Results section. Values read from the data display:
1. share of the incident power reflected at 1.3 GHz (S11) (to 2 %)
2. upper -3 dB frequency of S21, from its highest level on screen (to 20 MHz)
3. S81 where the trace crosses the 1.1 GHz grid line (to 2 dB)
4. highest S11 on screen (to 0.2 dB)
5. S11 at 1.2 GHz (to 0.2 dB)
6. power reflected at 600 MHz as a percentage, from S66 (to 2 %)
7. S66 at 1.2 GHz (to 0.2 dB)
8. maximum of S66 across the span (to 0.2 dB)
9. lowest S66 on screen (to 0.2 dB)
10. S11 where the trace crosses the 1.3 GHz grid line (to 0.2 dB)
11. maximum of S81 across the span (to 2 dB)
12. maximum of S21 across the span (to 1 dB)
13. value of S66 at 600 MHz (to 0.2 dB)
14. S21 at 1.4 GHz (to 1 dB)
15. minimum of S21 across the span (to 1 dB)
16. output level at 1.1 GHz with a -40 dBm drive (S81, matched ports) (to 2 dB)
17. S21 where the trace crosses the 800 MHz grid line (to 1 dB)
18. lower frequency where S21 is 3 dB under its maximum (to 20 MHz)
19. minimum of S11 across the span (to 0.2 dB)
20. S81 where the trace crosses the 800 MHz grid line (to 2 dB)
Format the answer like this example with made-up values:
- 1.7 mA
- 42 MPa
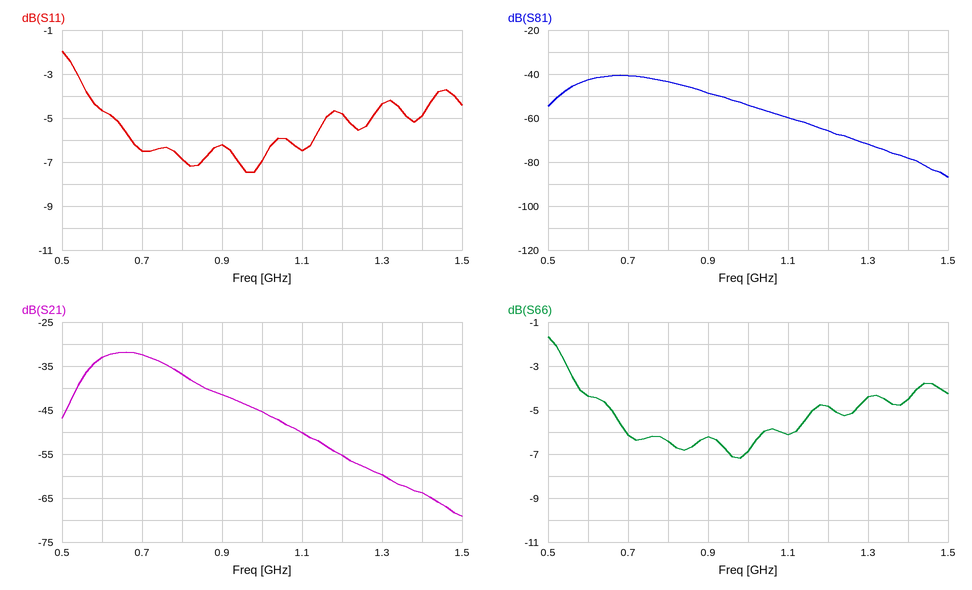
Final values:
- 36 %
- 760 MHz
- -60 dB
- -2.0 dB
- -4.8 dB
- 36 %
- -4.8 dB
- -1.6 dB
- -7.2 dB
- -4.4 dB
- -40 dB
- -32 dB
- -4.4 dB
- -64 dB
- -69 dB
- -100 dBm
- -37 dB
- 580 MHz
- -7.4 dB
- -44 dB
